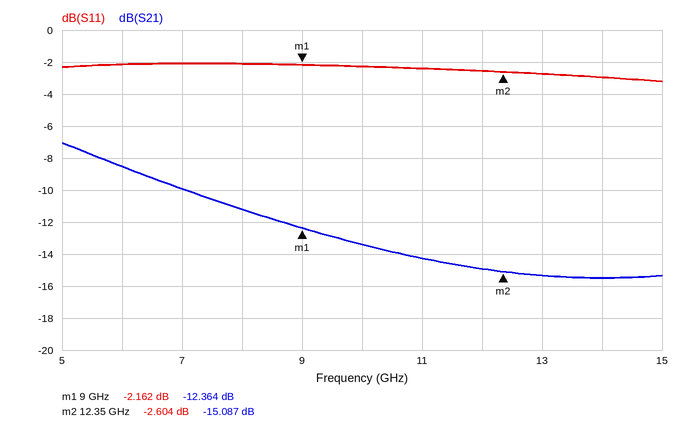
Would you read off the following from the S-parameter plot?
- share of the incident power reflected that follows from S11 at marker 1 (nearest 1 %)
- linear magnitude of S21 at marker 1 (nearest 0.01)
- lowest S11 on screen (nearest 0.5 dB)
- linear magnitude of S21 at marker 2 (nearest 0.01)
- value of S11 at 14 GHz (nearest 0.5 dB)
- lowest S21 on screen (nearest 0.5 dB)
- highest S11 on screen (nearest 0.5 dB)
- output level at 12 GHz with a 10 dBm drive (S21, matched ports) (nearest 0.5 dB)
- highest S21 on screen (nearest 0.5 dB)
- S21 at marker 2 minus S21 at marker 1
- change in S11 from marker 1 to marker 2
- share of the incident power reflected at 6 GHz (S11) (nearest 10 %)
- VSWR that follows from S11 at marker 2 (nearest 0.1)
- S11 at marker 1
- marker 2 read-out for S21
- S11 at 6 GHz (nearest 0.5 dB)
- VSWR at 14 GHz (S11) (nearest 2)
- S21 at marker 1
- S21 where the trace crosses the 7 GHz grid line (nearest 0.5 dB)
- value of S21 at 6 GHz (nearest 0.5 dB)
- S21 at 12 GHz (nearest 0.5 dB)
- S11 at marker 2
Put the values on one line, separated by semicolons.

61 %; 0.24; -3.0 dB; 0.18; -3.0 dB; -15.5 dB; -2.0 dB; -5.0 dBm; -7.0 dB; -2.723 dB; -0.442 dB; 60 %; 6.7; -2.162 dB; -15.087 dB; -2.0 dB; 6; -12.364 dB; -10.0 dB; -8.5 dB; -15.0 dB; -2.604 dB
